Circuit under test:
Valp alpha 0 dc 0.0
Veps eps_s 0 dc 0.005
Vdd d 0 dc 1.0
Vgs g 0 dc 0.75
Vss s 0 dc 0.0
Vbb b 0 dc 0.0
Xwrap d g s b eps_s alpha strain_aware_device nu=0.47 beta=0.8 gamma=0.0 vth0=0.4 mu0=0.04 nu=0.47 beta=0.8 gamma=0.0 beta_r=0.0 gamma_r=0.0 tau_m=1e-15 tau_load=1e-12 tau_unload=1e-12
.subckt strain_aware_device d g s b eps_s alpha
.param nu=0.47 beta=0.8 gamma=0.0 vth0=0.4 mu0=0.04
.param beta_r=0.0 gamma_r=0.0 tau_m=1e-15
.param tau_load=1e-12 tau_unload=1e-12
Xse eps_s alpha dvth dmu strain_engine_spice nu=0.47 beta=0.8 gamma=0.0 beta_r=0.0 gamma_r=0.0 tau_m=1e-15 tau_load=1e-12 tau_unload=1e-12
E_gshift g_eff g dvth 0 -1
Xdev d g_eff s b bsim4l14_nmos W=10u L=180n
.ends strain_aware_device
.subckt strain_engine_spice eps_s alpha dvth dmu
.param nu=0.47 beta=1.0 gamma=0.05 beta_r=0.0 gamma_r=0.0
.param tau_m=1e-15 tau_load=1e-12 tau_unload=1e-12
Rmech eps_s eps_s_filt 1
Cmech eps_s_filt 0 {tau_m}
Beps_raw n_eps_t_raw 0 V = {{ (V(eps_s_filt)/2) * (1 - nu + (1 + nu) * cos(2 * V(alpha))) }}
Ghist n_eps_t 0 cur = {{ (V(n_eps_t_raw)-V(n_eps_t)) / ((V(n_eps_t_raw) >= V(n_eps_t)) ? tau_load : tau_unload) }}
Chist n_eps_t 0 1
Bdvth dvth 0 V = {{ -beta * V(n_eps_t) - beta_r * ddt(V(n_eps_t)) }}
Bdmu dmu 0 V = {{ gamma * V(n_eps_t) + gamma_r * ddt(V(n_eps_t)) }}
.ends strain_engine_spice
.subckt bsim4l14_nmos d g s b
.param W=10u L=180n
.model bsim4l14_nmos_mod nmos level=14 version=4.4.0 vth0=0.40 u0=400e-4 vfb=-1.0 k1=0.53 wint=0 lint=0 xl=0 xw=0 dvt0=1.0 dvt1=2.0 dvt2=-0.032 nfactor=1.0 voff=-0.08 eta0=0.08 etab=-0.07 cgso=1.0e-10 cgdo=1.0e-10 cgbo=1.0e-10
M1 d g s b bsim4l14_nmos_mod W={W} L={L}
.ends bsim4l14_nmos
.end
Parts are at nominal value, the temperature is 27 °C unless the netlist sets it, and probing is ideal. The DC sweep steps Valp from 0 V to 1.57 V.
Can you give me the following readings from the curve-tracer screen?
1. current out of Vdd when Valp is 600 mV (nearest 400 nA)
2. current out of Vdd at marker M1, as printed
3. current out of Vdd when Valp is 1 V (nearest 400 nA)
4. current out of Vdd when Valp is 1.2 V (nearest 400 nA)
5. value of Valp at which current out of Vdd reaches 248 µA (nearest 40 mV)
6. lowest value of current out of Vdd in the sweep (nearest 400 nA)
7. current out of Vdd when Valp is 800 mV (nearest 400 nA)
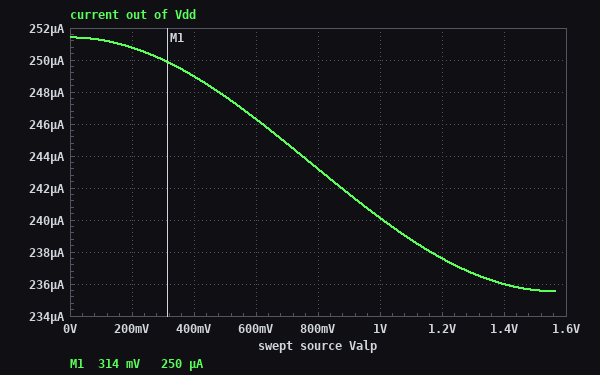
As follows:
246.4 µA
250 µA
240.0 µA
237.6 µA
480 mV
235.6 µA
243.2 µA
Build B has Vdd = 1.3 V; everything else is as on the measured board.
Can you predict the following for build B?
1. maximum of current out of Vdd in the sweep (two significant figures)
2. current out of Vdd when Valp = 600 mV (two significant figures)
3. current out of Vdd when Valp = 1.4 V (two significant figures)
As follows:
280 µA
270 µA
260 µA
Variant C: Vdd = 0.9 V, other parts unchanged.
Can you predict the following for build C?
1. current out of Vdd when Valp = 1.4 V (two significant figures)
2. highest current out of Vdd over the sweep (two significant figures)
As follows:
230 µA
240 µA
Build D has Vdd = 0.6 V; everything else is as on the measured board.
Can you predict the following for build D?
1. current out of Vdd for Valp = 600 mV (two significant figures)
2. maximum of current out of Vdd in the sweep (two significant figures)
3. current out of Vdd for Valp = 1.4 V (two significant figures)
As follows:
210 µA
220 µA
200 µA
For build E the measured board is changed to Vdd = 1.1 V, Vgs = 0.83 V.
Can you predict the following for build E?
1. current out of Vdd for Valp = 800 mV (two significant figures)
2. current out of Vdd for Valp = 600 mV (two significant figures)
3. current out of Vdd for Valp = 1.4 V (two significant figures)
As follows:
500 µA
510 µA
490 µA
